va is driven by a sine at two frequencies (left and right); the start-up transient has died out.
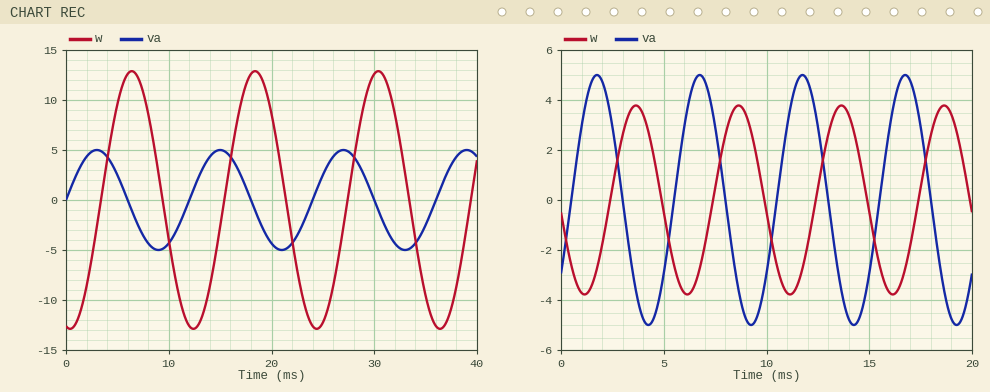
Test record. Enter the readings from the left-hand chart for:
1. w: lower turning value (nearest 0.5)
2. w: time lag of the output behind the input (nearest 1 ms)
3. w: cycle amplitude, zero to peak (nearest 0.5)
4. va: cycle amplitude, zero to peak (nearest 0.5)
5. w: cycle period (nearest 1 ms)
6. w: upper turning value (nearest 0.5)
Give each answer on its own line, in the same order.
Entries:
-13.0
3 ms
13.0
5.0
12 ms
13.0
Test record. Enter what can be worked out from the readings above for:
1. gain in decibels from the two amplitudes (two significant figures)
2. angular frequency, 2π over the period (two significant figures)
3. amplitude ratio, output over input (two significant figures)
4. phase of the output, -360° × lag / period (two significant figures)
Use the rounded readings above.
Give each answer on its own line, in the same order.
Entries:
8.3 dB
0.52 rad/ms
2.6
-90°
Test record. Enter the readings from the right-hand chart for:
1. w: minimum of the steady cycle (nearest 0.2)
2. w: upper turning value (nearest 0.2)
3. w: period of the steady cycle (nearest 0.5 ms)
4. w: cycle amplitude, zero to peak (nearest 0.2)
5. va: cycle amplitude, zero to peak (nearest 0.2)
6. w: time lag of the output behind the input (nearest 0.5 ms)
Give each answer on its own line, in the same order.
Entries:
-3.8
3.8
5.0 ms
3.8
5.0
2.0 ms
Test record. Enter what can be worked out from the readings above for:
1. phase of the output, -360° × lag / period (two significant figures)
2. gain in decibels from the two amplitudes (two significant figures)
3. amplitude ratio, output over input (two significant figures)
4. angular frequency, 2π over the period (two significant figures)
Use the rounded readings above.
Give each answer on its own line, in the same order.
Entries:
-140°
-2.4 dB
0.76
1.3 rad/ms
